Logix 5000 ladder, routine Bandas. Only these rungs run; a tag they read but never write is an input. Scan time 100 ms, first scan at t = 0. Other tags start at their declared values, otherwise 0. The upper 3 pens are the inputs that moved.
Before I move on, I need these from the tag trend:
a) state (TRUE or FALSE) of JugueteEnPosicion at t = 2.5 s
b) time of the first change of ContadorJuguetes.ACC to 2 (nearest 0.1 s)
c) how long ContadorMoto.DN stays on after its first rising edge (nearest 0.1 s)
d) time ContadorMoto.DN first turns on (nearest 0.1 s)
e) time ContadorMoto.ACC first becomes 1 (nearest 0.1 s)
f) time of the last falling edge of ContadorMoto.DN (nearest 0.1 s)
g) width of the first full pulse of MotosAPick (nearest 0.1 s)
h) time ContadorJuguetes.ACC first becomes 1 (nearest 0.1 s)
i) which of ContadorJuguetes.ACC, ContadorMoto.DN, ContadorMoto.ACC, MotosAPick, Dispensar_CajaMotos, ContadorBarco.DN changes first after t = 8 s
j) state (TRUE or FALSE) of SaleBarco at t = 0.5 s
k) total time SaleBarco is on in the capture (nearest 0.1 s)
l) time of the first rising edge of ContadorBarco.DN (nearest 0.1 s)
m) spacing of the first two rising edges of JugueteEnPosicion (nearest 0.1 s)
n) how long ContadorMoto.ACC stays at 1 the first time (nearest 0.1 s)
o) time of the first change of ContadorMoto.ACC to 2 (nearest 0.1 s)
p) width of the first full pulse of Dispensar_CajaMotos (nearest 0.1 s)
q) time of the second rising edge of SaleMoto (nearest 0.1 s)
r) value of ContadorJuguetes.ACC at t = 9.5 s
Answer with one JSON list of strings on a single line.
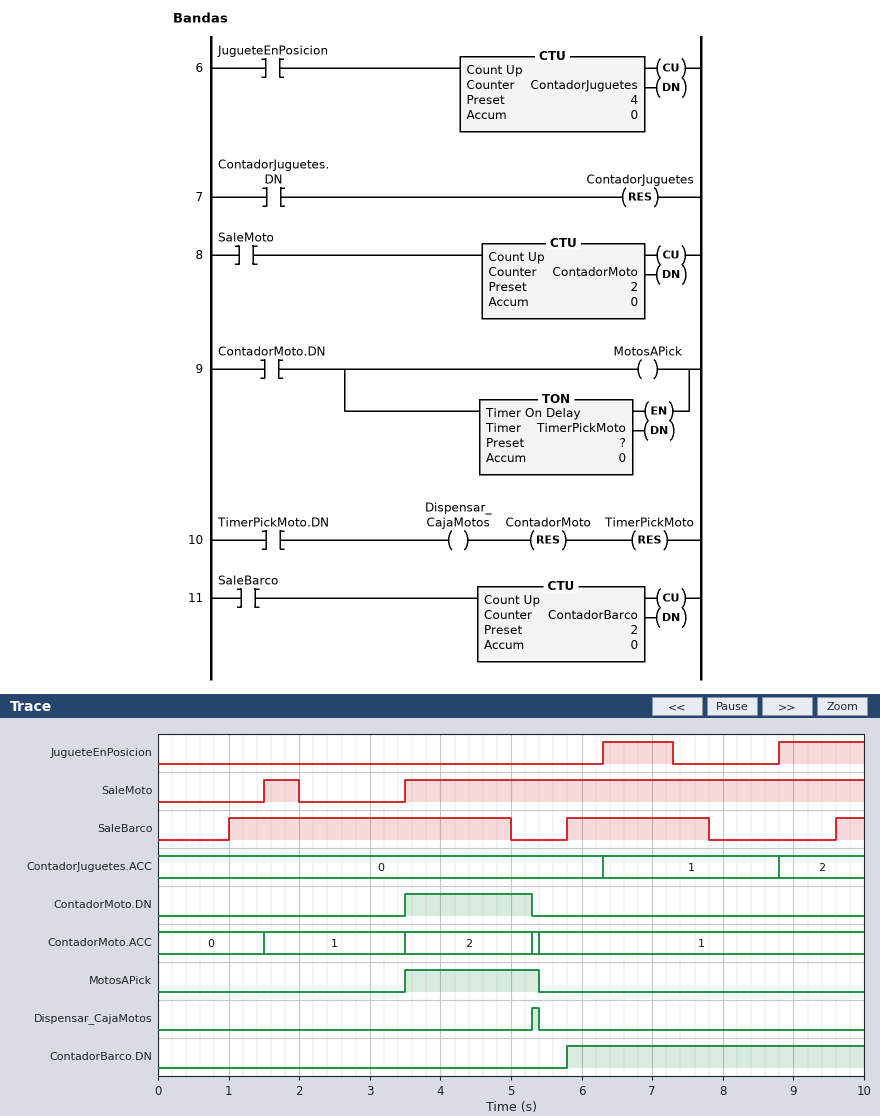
["FALSE", "8.8 s", "1.8 s", "3.5 s", "1.5 s", "5.3 s", "1.9 s", "6.3 s", "ContadorJuguetes.ACC", "FALSE", "6.4 s", "5.8 s", "2.5 s", "2.0 s", "3.5 s", "0.1 s", "3.5 s", "2"]
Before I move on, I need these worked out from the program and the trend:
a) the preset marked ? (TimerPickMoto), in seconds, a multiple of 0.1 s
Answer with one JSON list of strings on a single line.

["1.8 s"]
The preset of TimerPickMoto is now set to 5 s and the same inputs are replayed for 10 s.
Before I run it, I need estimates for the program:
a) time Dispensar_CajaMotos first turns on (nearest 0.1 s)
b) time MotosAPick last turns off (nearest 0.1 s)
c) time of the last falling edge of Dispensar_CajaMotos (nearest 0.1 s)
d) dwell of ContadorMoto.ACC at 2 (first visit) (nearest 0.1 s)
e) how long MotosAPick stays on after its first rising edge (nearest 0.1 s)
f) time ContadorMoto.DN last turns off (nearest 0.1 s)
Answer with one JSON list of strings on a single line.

["8.5 s", "8.6 s", "8.6 s", "5.0 s", "5.1 s", "8.5 s"]
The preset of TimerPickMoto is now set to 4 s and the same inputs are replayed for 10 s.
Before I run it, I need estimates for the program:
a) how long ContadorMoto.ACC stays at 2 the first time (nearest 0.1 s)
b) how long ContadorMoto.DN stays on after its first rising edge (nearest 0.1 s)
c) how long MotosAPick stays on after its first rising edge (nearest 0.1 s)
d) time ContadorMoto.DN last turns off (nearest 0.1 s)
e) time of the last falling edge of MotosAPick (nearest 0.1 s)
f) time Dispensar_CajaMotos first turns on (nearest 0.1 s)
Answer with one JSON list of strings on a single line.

["4.0 s", "4.0 s", "4.1 s", "7.5 s", "7.6 s", "7.5 s"]
